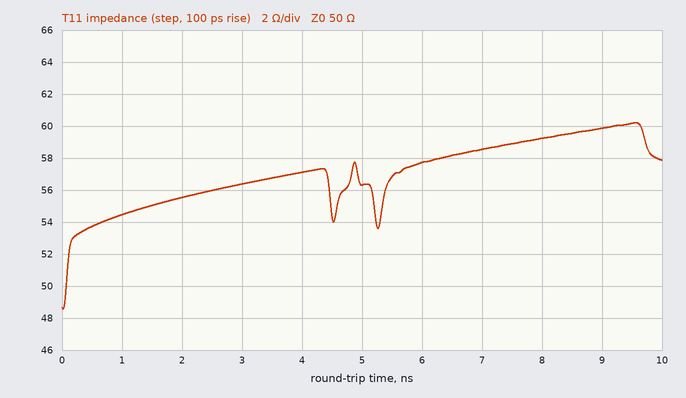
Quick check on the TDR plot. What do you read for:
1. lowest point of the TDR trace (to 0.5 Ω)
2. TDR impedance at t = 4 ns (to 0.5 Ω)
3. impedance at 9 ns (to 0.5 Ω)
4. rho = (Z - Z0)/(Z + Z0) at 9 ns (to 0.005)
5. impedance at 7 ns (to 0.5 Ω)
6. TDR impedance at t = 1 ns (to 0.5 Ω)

48.5 Ω
57.0 Ω
60.0 Ω
+0.090
58.5 Ω
54.5 Ω
